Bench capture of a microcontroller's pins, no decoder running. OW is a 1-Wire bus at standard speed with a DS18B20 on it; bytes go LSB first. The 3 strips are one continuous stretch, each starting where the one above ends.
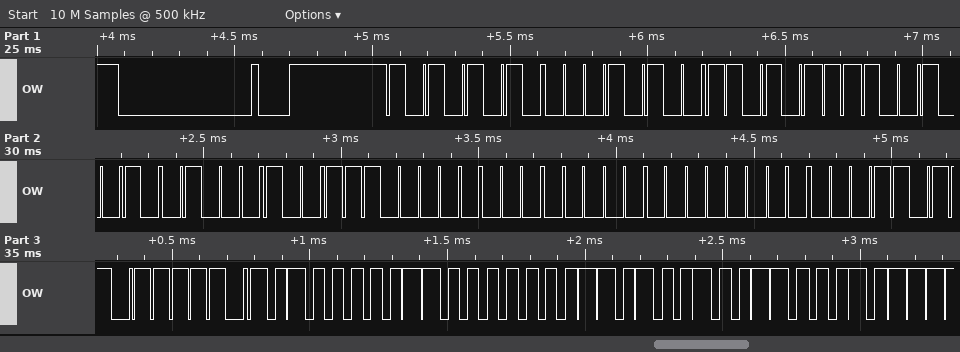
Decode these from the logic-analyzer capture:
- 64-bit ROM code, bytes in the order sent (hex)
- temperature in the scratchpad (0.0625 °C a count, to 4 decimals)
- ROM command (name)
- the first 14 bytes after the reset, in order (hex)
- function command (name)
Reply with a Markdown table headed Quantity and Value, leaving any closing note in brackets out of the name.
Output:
| Quantity | Value |
|---|---|
| 64-bit ROM code, bytes in the order sent | 28 EB 49 22 07 00 00 D8 |
| temperature in the scratchpad | 24.1250 °C |
| ROM command | Match ROM |
| the first 14 bytes after the reset, in order | 55 28 EB 49 22 07 00 00 D8 BE 82 01 4B 46 |
| function command | Read Scratchpad |
